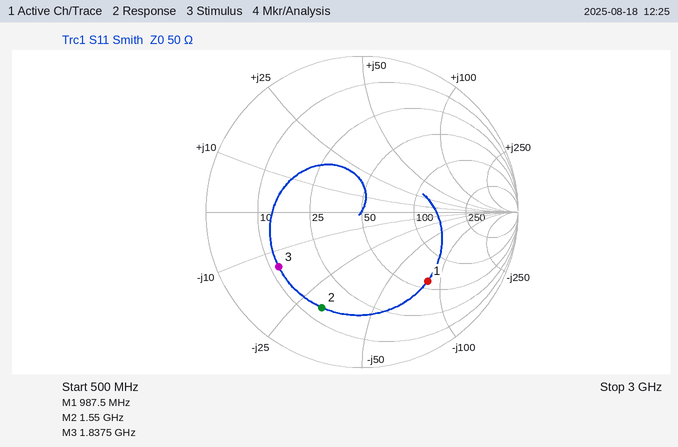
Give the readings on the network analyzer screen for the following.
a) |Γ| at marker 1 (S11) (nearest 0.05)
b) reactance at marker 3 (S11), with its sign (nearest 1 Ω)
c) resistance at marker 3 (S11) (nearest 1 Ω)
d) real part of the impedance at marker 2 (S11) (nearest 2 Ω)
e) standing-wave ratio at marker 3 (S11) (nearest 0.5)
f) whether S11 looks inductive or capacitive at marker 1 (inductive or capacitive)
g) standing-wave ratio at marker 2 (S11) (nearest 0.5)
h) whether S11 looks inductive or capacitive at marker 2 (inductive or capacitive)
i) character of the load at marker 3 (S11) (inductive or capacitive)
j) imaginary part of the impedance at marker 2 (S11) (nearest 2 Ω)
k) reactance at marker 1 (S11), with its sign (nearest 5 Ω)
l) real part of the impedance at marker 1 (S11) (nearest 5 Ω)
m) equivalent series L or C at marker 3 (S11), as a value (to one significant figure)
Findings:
0.60
-14 Ω
12 Ω
14 Ω
4.5
capacitive
5.0
capacitive
capacitive
-32 Ω
-85 Ω
60 Ω
6 pF
